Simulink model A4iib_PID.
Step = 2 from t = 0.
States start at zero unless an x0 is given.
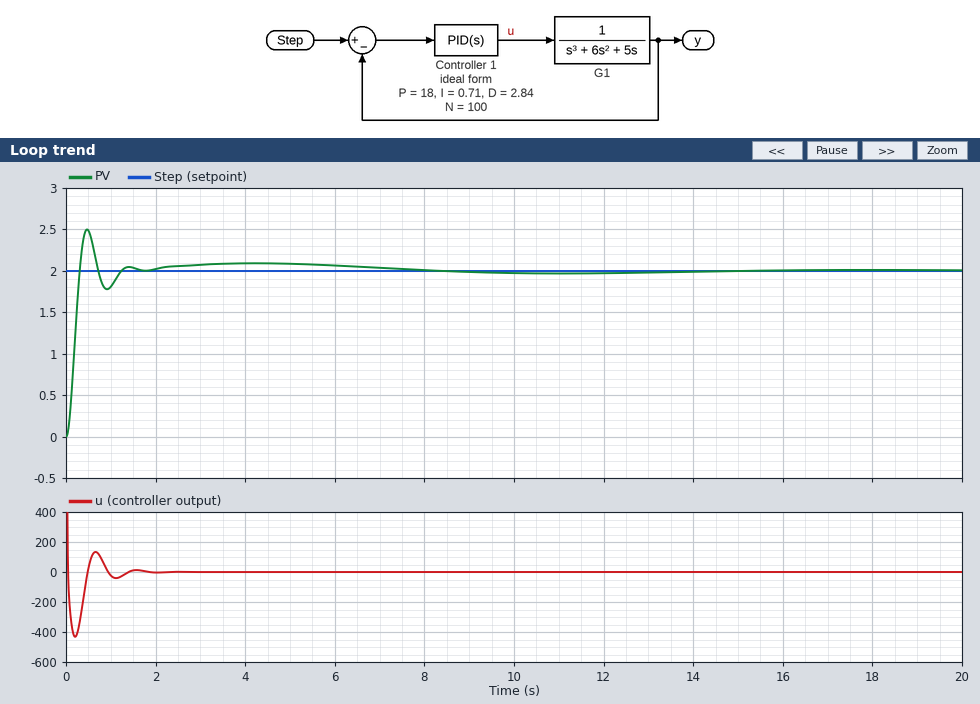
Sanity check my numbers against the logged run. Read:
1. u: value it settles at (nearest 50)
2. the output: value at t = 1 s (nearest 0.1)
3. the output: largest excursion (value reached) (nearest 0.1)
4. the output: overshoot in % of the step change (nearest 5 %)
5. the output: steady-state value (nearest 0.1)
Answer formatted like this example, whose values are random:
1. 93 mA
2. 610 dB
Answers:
1. 0
2. 1.8
3. 2.5
4. 25 %
5. 2.0
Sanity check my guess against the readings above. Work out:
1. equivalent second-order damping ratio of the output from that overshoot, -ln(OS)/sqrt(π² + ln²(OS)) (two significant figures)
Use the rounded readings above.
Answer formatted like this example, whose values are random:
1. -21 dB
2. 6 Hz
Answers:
1. 0.40
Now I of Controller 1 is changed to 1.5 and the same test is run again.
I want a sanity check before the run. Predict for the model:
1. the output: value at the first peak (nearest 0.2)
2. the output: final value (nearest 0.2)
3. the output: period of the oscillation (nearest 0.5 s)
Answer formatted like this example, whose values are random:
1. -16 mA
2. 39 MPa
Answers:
1. 2.6
2. 2.0
3. 2.5 s
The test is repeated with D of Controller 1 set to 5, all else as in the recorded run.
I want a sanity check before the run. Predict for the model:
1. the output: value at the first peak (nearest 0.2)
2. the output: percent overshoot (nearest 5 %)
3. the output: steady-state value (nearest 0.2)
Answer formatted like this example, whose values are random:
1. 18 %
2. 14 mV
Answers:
1. 2.8
2. 40 %
3. 2.0
